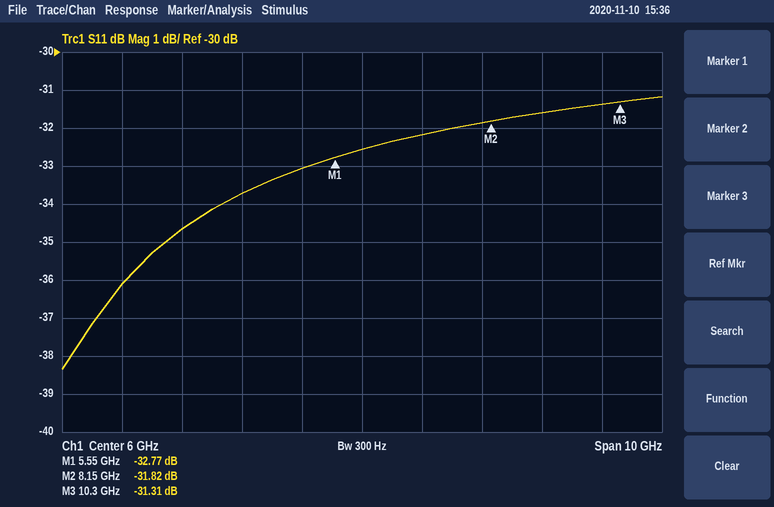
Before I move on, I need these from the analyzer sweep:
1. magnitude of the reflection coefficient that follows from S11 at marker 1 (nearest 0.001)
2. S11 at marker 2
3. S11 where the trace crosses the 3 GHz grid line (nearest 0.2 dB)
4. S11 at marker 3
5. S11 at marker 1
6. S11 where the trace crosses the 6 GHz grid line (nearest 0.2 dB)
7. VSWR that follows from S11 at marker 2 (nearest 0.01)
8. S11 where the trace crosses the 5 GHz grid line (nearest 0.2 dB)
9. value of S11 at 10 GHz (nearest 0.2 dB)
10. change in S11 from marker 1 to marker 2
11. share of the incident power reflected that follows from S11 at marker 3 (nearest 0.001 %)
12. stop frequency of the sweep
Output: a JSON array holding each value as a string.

["0.023", "-31.82 dB", "-34.6 dB", "-31.31 dB", "-32.77 dB", "-32.6 dB", "1.05", "-33.0 dB", "-31.4 dB", "0.95 dB", "0.074 %", "11 GHz"]
